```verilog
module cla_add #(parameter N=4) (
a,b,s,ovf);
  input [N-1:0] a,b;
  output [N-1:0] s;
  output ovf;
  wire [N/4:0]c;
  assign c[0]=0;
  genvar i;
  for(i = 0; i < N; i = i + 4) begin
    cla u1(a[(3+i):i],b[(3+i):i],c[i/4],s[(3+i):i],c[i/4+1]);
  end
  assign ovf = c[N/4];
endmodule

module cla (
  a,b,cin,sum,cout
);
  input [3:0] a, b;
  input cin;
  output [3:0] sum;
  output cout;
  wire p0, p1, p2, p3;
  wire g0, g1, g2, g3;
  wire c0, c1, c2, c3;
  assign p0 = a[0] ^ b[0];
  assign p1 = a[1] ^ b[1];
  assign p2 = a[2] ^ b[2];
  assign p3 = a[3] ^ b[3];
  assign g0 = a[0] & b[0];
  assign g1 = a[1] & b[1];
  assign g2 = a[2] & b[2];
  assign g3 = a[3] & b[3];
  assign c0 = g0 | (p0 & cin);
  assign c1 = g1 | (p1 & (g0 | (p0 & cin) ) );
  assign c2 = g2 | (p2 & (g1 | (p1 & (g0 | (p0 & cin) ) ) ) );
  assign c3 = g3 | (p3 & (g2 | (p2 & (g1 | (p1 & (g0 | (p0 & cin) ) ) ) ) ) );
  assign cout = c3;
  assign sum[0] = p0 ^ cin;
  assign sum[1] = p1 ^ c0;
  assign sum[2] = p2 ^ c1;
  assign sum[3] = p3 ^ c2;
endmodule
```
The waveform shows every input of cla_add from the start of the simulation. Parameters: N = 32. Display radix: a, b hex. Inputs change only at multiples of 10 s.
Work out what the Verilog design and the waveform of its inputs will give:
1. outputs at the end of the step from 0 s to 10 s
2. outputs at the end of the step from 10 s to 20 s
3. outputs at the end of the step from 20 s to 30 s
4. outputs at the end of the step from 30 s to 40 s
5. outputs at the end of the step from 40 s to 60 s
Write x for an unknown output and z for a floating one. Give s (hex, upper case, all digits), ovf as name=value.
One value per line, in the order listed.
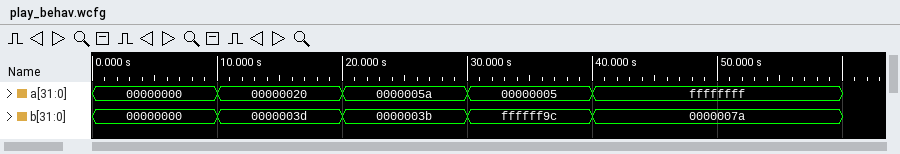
s=00000000, ovf=0
s=0000005D, ovf=0
s=00000095, ovf=0
s=FFFFFFA1, ovf=0
s=00000079, ovf=1
